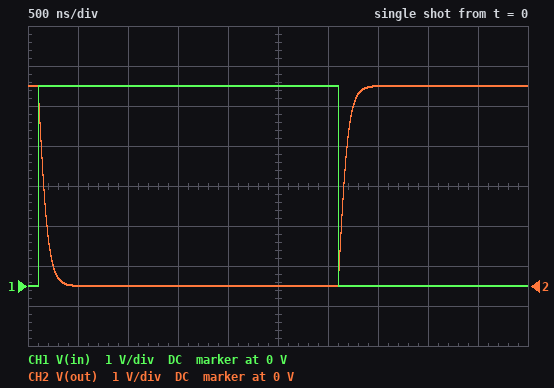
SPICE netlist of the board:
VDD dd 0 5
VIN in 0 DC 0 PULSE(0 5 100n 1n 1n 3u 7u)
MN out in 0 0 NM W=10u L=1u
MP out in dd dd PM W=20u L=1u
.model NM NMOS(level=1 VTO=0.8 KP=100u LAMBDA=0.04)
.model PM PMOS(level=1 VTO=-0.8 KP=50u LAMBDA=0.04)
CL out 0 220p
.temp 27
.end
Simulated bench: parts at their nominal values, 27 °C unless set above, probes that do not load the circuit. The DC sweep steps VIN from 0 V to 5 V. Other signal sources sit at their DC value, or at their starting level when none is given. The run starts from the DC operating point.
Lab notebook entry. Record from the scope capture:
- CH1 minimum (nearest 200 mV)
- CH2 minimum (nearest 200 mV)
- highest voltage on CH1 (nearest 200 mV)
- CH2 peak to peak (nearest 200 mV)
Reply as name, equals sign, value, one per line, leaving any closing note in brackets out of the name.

CH1 minimum = 0 V
CH2 minimum = 0 V
highest voltage on CH1 = 5.0 V
CH2 peak to peak = 5.0 V
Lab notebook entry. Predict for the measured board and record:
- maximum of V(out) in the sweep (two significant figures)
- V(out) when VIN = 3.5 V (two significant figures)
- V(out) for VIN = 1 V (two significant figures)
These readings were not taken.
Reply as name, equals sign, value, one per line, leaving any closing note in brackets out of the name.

maximum of V(out) in the sweep = 5.0 V
V(out) when VIN = 3.5 V = 110 mV
V(out) for VIN = 1 V = 5.0 V
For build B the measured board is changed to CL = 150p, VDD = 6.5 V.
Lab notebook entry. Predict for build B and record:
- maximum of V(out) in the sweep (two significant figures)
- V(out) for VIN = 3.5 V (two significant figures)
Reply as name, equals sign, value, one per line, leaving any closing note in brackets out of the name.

maximum of V(out) in the sweep = 6.5 V
V(out) for VIN = 3.5 V = 1.4 V
